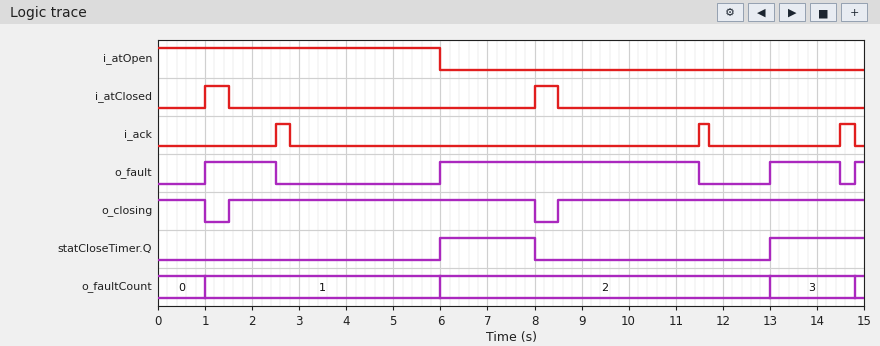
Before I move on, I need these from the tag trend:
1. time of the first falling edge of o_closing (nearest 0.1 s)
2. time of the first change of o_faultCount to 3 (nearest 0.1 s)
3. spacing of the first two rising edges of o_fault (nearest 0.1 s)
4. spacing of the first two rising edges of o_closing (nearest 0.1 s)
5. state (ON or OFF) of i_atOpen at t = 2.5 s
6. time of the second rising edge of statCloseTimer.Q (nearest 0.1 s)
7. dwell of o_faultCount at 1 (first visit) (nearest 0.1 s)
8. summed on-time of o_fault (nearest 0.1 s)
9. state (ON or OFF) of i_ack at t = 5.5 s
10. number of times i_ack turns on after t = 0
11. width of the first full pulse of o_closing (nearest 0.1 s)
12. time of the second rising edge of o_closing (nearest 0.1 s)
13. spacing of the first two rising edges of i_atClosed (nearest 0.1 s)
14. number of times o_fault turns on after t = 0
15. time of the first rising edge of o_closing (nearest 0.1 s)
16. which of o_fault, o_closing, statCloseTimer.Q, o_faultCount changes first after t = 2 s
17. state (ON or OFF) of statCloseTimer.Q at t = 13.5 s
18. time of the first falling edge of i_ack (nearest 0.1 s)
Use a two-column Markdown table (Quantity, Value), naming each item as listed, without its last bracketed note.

| Quantity | Value |
|---|---|
| time of the first falling edge of o_closing | 1.0 s |
| time of the first change of o_faultCount to 3 | 13.0 s |
| spacing of the first two rising edges of o_fault | 5.0 s |
| spacing of the first two rising edges of o_closing | 7.0 s |
| state (ON or OFF) of i_atOpen at t = 2.5 s | ON |
| time of the second rising edge of statCloseTimer.Q | 13.0 s |
| dwell of o_faultCount at 1 (first visit) | 5.0 s |
| summed on-time of o_fault | 8.7 s |
| state (ON or OFF) of i_ack at t = 5.5 s | OFF |
| number of times i_ack turns on after t = 0 | 3 |
| width of the first full pulse of o_closing | 6.5 s |
| time of the second rising edge of o_closing | 8.5 s |
| spacing of the first two rising edges of i_atClosed | 7.0 s |
| number of times o_fault turns on after t = 0 | 4 |
| time of the first rising edge of o_closing | 1.5 s |
| which of o_fault, o_closing, statCloseTimer.Q, o_faultCount changes first after t = 2 s | o_fault |
| state (ON or OFF) of statCloseTimer.Q at t = 13.5 s | ON |
| time of the first falling edge of i_ack | 2.8 s |
